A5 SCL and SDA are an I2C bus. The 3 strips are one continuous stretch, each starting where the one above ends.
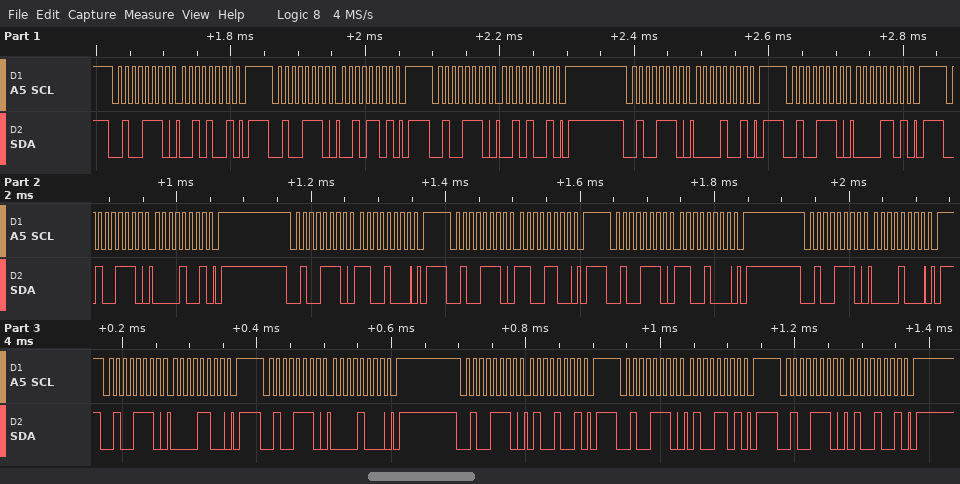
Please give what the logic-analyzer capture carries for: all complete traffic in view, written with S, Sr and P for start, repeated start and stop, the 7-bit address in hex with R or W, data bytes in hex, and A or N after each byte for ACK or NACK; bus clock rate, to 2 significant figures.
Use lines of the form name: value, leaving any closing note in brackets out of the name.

all complete traffic in view, written with S, Sr and P for start, repeated start and stop, the 7-bit address in hex with R or W, data bytes in hex, and A or N after each byte for ACK or NACK: S 27W A 29 A P S 27W A 2D A P S 27W A 29 A P S 27W A 09 A P S 27W A 0D A P S 27W A 09 A P S 27W A C8 A P S 27W A CC A P S 27W A C8 A P S 27W A 08 A P S 27W A 0C A P S 27W A 08 A P S 27W A 49 A P S 27W A 4D A P S 27W A 49 A P
bus clock rate, to 2 significant figures: 100 kHz
